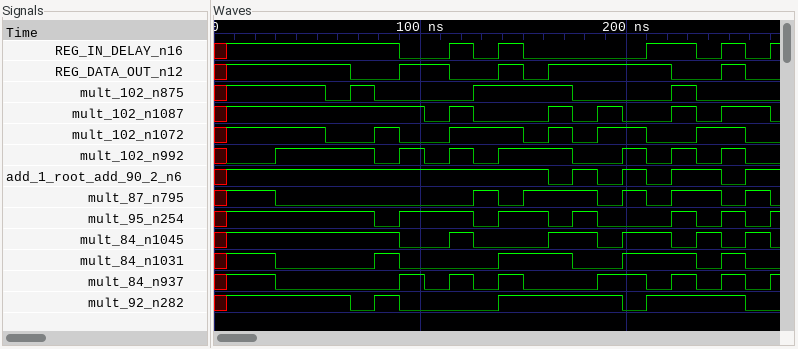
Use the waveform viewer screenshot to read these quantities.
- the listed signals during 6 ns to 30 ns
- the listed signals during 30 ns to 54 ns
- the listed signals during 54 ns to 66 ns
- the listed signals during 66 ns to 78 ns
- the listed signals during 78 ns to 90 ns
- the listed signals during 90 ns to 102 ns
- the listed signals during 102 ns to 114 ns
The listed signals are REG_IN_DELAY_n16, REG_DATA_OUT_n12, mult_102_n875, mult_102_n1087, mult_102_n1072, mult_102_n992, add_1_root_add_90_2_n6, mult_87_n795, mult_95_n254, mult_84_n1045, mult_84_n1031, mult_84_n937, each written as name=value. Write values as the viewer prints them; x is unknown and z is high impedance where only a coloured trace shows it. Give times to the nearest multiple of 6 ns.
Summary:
REG_IN_DELAY_n16=1, REG_DATA_OUT_n12=1, mult_102_n875=1, mult_102_n1087=1, mult_102_n1072=1, mult_102_n992=0, add_1_root_add_90_2_n6=1, mult_87_n795=1, mult_95_n254=1, mult_84_n1045=1, mult_84_n1031=1, mult_84_n937=1
REG_IN_DELAY_n16=1, REG_DATA_OUT_n12=1, mult_102_n875=1, mult_102_n1087=1, mult_102_n1072=1, mult_102_n992=1, add_1_root_add_90_2_n6=1, mult_87_n795=0, mult_95_n254=1, mult_84_n1045=1, mult_84_n1031=0, mult_84_n937=0
REG_IN_DELAY_n16=1, REG_DATA_OUT_n12=1, mult_102_n875=0, mult_102_n1087=1, mult_102_n1072=0, mult_102_n992=1, add_1_root_add_90_2_n6=1, mult_87_n795=0, mult_95_n254=1, mult_84_n1045=1, mult_84_n1031=0, mult_84_n937=0
REG_IN_DELAY_n16=1, REG_DATA_OUT_n12=0, mult_102_n875=1, mult_102_n1087=1, mult_102_n1072=0, mult_102_n992=1, add_1_root_add_90_2_n6=1, mult_87_n795=0, mult_95_n254=1, mult_84_n1045=1, mult_84_n1031=0, mult_84_n937=0
REG_IN_DELAY_n16=1, REG_DATA_OUT_n12=0, mult_102_n875=0, mult_102_n1087=1, mult_102_n1072=1, mult_102_n992=0, add_1_root_add_90_2_n6=1, mult_87_n795=0, mult_95_n254=0, mult_84_n1045=1, mult_84_n1031=1, mult_84_n937=0
REG_IN_DELAY_n16=0, REG_DATA_OUT_n12=1, mult_102_n875=0, mult_102_n1087=1, mult_102_n1072=0, mult_102_n992=1, add_1_root_add_90_2_n6=1, mult_87_n795=0, mult_95_n254=1, mult_84_n1045=0, mult_84_n1031=0, mult_84_n937=1
REG_IN_DELAY_n16=0, REG_DATA_OUT_n12=1, mult_102_n875=0, mult_102_n1087=0, mult_102_n1072=0, mult_102_n992=0, add_1_root_add_90_2_n6=1, mult_87_n795=0, mult_95_n254=1, mult_84_n1045=0, mult_84_n1031=0, mult_84_n937=0
